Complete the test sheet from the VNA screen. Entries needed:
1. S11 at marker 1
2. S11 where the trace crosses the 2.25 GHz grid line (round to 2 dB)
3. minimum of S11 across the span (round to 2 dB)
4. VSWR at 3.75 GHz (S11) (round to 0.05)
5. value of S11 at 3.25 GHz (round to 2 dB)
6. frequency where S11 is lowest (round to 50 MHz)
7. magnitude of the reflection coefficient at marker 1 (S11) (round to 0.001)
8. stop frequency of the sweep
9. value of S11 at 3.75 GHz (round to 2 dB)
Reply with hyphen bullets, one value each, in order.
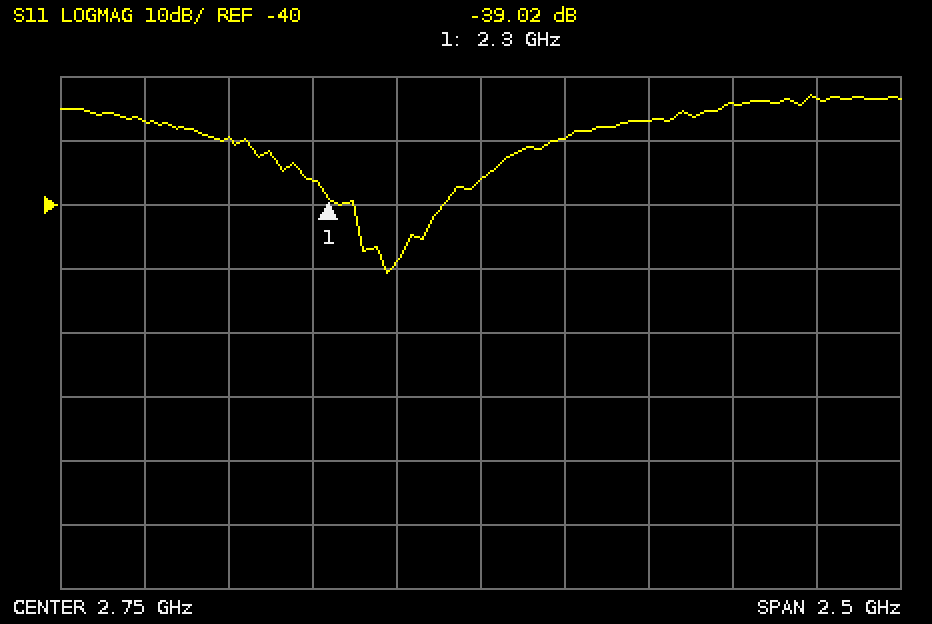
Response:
- -39.02 dB
- -36 dB
- -50 dB
- 1.15
- -26 dB
- 2.45 GHz
- 0.011
- 4 GHz
- -24 dB
